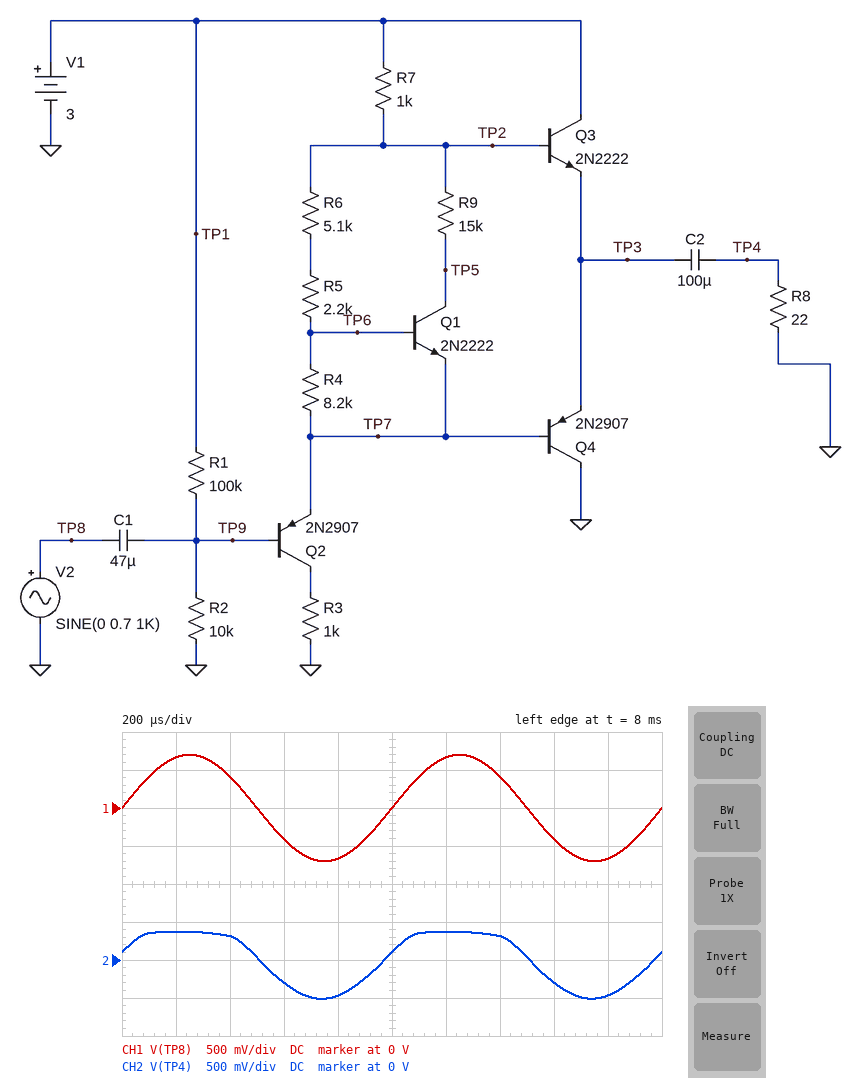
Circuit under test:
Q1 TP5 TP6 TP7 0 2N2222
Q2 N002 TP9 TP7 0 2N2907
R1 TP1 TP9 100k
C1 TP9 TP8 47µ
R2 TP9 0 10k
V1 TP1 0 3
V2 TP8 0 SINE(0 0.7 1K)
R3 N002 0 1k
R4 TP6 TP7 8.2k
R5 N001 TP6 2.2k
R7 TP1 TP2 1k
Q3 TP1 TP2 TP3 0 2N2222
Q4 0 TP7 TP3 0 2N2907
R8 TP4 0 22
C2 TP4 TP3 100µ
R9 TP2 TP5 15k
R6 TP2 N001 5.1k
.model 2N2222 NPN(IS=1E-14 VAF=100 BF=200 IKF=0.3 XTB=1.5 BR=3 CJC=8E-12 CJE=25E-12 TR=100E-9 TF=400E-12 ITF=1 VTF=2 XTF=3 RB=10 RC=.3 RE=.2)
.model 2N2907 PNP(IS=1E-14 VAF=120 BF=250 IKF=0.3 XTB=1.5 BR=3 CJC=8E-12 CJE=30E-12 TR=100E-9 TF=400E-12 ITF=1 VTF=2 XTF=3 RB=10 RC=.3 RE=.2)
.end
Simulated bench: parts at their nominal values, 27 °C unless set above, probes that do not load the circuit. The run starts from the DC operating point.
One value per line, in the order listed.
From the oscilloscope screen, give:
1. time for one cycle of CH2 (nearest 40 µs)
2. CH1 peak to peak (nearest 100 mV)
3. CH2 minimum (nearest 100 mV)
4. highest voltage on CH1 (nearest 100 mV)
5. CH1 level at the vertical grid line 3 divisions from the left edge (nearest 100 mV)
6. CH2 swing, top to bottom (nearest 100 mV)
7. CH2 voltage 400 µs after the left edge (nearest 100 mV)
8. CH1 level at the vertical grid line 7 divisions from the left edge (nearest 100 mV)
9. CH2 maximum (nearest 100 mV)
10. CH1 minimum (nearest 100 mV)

1.00 ms
1.4 V
-500 mV
700 mV
-400 mV
900 mV
300 mV
400 mV
400 mV
-700 mV
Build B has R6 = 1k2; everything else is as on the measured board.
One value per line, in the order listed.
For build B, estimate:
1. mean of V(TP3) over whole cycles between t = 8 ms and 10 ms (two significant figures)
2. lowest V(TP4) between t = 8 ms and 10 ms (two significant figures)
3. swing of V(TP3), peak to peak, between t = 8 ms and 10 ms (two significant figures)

1.6 V
-490 mV
840 mV
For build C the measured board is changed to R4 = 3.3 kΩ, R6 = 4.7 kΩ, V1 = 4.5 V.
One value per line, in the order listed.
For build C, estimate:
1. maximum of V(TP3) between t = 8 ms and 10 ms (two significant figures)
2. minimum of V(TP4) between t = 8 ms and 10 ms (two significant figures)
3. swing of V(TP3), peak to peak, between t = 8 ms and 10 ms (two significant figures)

2.8 V
-600 mV
1.2 V
